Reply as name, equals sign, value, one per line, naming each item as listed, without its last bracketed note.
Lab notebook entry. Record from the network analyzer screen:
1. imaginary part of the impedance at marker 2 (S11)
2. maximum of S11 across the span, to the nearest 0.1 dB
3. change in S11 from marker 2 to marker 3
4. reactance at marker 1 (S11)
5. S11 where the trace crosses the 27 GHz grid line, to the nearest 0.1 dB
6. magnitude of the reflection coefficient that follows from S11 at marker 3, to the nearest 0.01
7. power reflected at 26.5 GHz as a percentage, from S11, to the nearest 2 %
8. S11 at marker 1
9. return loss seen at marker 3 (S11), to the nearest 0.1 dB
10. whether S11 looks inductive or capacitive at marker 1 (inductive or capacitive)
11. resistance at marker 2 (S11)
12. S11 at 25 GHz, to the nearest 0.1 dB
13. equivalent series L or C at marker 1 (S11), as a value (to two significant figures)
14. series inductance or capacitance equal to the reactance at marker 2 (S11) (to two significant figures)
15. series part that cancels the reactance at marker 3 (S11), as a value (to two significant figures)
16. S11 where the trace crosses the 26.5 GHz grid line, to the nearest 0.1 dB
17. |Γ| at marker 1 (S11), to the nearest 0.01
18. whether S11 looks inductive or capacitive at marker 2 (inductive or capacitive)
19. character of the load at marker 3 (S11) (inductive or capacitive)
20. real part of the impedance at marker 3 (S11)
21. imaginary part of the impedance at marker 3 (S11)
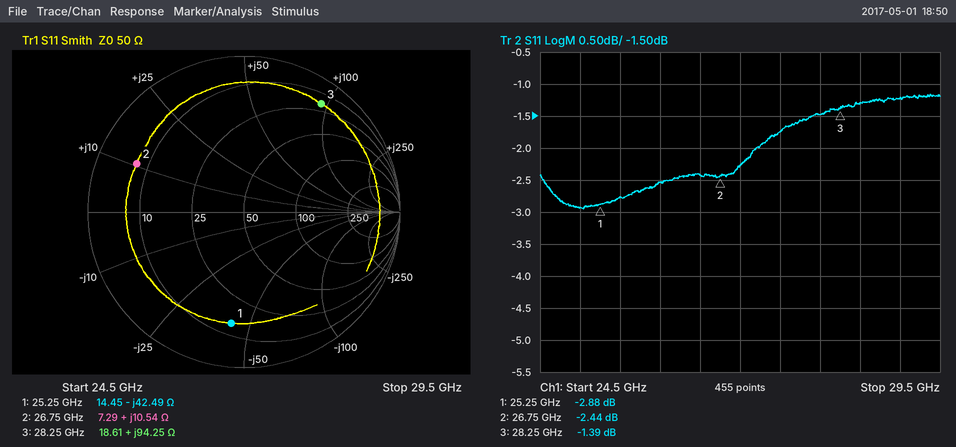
imaginary part of the impedance at marker 2 = +10.54 Ω
maximum of S11 across the span, to the nearest 0.1 dB = -1.2 dB
change in S11 from marker 2 to marker 3 = 1.05 dB
reactance at marker 1 = -42.49 Ω
S11 where the trace crosses the 27 GHz grid line, to the nearest 0.1 dB = -2.3 dB
magnitude of the reflection coefficient that follows from S11 at marker 3, to the nearest 0.01 = 0.85
power reflected at 26.5 GHz as a percentage, from S11, to the nearest 2 % = 58 %
S11 at marker 1 = -2.88 dB
return loss seen at marker 3 (S11), to the nearest 0.1 dB = 1.4 dB
whether S11 looks inductive or capacitive at marker 1 = capacitive
resistance at marker 2 = 7.29 Ω
S11 at 25 GHz, to the nearest 0.1 dB = -2.9 dB
equivalent series L or C at marker 1 (S11), as a value = 150 fF
series inductance or capacitance equal to the reactance at marker 2 (S11) = 63 pH
series part that cancels the reactance at marker 3 (S11), as a value = 60 fF
S11 where the trace crosses the 26.5 GHz grid line, to the nearest 0.1 dB = -2.4 dB
|Γ| at marker 1 (S11), to the nearest 0.01 = 0.72
whether S11 looks inductive or capacitive at marker 2 = inductive
character of the load at marker 3 (S11) = inductive
real part of the impedance at marker 3 = 18.61 Ω
imaginary part of the impedance at marker 3 = +94.25 Ω
